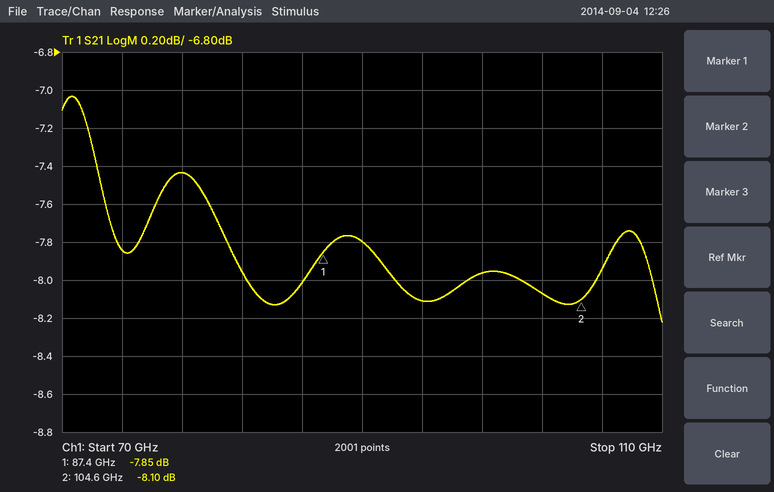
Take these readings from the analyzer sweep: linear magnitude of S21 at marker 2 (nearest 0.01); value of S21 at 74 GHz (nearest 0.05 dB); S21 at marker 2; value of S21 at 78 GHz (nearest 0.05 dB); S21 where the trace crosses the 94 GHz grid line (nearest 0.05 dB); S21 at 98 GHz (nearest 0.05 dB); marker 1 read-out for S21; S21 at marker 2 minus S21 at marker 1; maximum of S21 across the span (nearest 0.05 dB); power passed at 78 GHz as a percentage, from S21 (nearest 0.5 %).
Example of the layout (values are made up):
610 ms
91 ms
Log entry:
0.39
-7.85 dB
-8.10 dB
-7.45 dB
-8.10 dB
-7.95 dB
-7.85 dB
-0.25 dB
-7.05 dB
18.0 %
